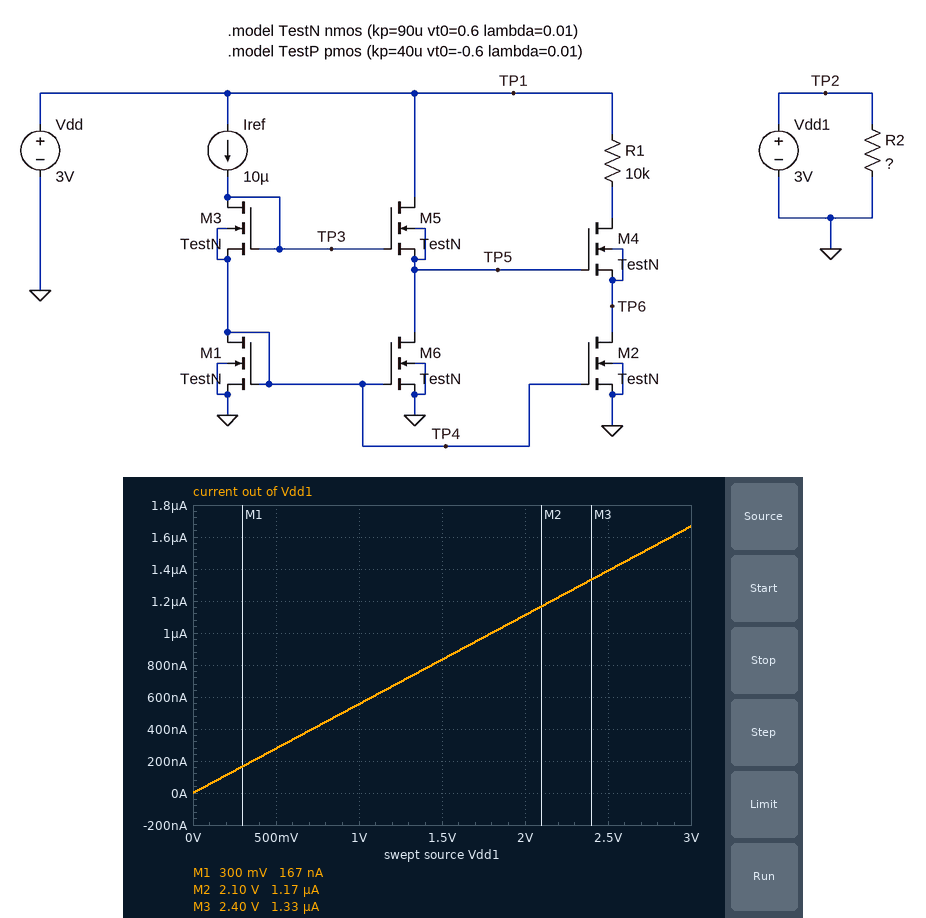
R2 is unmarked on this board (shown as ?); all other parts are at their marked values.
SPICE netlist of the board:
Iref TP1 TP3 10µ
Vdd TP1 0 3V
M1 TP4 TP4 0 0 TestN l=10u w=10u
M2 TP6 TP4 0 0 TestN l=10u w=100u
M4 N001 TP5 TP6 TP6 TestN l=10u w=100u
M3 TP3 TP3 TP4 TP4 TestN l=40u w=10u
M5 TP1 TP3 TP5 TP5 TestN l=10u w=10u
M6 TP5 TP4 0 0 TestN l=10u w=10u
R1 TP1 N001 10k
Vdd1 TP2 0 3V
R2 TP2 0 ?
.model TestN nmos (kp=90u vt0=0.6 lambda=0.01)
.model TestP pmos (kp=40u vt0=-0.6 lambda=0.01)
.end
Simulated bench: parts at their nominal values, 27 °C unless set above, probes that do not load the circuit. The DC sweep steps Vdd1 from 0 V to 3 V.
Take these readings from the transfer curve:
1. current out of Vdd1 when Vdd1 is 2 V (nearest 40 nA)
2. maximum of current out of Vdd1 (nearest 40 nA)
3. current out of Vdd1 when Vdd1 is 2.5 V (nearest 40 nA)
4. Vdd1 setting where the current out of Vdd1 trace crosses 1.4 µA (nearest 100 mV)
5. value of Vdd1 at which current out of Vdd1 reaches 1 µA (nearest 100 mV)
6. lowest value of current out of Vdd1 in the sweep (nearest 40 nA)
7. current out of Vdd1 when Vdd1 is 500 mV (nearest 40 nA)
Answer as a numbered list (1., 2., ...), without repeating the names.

1. 1.12 µA
2. 1.68 µA
3. 1.40 µA
4. 2.5 V
5. 1.8 V
6. 0 A
7. 280 nA
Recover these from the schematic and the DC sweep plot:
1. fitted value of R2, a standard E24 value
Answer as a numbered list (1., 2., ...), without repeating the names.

1. 1.8 MΩ
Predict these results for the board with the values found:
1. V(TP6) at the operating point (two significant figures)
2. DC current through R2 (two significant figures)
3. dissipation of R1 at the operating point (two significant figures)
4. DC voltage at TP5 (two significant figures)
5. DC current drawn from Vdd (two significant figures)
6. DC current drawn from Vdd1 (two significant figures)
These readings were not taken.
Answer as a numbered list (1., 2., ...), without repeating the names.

1. 470 mV
2. 1.7 µA
3. 99 µW
4. 1.5 V
5. 120 µA
6. 1.7 µA
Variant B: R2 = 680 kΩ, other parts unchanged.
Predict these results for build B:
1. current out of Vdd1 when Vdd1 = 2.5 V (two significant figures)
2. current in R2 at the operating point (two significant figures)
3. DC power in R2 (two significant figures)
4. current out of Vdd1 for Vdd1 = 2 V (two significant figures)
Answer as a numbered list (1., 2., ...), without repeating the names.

1. 3.7 µA
2. 4.4 µA
3. 13 µW
4. 2.9 µA
